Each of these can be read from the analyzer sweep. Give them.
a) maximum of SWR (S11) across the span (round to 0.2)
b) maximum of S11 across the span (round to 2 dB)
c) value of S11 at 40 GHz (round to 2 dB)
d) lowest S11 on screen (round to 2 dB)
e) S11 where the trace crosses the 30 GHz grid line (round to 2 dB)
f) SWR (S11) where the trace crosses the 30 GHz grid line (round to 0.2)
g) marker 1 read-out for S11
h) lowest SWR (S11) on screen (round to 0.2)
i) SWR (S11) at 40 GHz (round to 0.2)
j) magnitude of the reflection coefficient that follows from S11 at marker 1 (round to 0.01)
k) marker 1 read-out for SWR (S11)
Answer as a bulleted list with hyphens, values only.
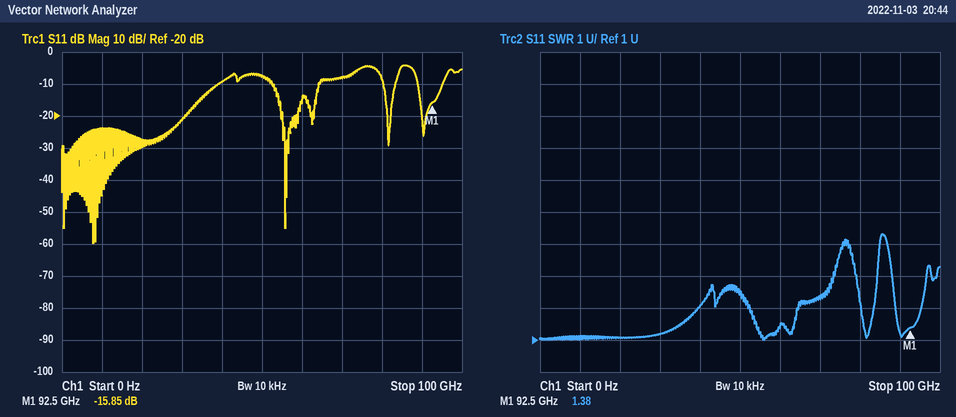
- 4.4
- -4 dB
- -10 dB
- -60 dB
- -22 dB
- 1.2
- -15.85 dB
- 1.0
- 2.0
- 0.16
- 1.38
